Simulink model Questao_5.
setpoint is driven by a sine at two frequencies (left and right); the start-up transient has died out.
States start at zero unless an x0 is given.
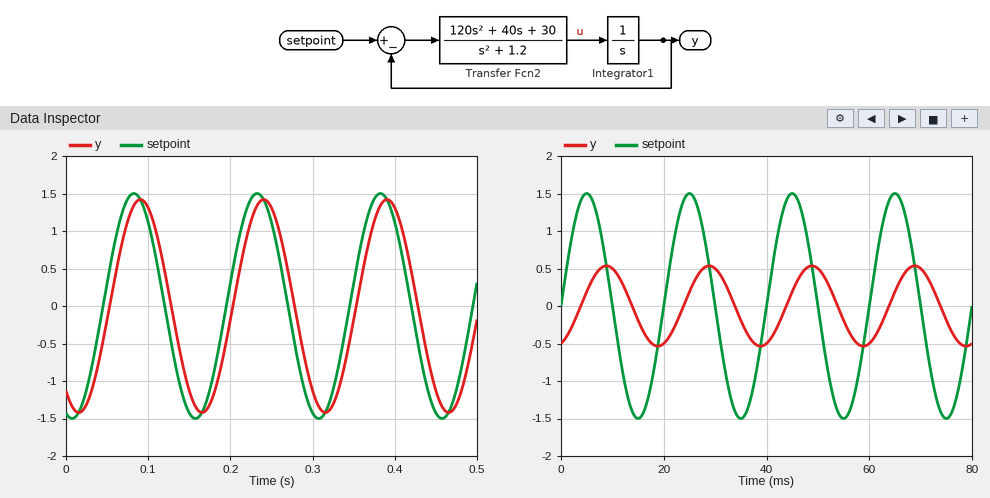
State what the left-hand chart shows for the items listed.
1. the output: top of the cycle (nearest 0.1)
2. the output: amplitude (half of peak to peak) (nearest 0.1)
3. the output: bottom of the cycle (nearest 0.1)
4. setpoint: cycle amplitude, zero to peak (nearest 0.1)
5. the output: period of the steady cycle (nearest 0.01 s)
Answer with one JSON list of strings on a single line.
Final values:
["1.4", "1.4", "-1.4", "1.5", "0.15 s"]
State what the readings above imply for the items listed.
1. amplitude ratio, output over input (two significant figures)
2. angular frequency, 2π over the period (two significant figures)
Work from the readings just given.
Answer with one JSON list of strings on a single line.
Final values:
["0.93", "42 rad/s"]
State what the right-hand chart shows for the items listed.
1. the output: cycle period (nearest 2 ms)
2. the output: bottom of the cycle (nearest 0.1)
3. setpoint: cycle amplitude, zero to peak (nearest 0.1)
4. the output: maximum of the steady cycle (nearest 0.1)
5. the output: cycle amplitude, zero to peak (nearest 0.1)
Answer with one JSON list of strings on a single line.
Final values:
["20 ms", "-0.5", "1.5", "0.5", "0.5"]
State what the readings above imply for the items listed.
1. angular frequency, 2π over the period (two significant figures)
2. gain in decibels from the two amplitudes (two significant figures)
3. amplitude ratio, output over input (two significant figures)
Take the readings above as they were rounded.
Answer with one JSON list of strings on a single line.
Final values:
["0.31 rad/ms", "-9.5 dB", "0.33"]
